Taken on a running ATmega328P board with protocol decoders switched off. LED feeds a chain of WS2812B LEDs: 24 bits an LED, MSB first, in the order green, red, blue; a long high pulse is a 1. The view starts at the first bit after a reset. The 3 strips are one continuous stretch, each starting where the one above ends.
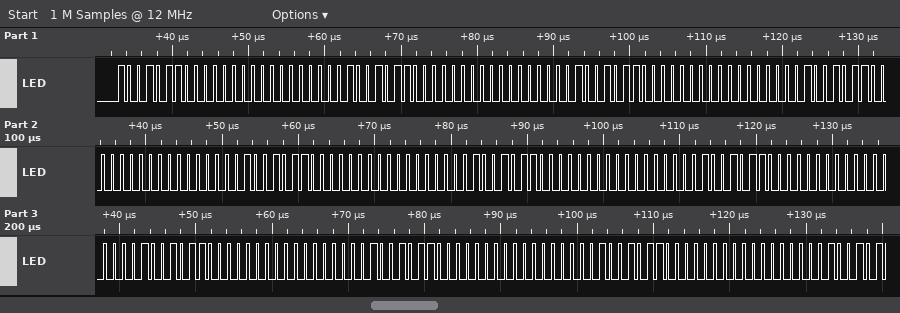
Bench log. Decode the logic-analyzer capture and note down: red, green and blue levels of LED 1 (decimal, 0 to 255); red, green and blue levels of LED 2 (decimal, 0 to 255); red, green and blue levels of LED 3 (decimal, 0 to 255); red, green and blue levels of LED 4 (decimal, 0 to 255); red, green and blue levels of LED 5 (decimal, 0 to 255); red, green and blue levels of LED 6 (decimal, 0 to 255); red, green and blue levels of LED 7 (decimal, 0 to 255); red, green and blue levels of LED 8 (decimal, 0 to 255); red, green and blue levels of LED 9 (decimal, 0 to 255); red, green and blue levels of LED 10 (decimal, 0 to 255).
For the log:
0, 150, 0
0, 150, 0
0, 150, 0
0, 150, 0
0, 150, 0
0, 150, 0
0, 150, 0
0, 150, 0
0, 150, 0
0, 150, 0
